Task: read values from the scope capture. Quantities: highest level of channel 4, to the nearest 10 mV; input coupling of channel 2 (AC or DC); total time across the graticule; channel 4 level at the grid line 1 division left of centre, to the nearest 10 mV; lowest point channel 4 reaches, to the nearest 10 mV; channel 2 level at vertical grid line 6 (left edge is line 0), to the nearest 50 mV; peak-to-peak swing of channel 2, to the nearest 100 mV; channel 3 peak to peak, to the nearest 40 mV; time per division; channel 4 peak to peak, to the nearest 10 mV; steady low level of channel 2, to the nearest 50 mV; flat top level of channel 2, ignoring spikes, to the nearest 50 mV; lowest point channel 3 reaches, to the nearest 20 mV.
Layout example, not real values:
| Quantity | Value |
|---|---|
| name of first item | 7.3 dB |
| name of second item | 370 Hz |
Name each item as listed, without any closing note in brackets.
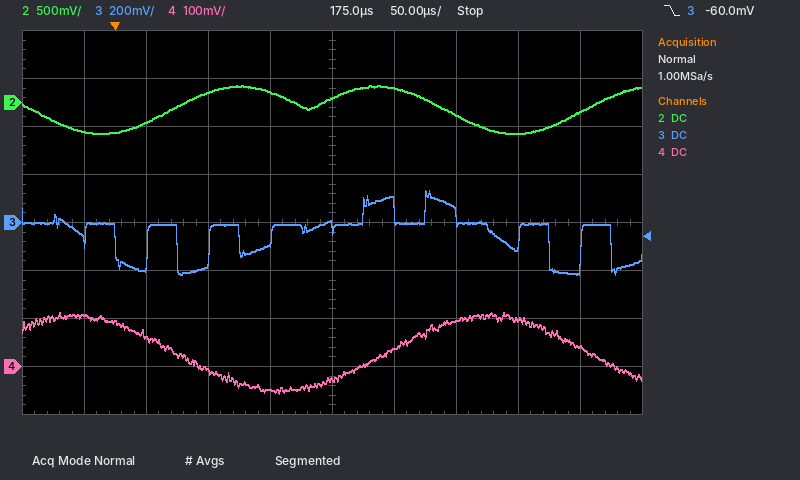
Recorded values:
| Quantity | Value |
|---|---|
| highest level of channel 4, to the nearest 10 mV | 110 mV |
| input coupling of channel 2 | DC |
| total time across the graticule | 500 µs |
| channel 4 level at the grid line 1 division left of centre, to the nearest 10 mV | -50 mV |
| lowest point channel 4 reaches, to the nearest 10 mV | -60 mV |
| channel 2 level at vertical grid line 6 (left edge is line 0), to the nearest 50 mV | 150 mV |
| peak-to-peak swing of channel 2, to the nearest 100 mV | 500 mV |
| channel 3 peak to peak, to the nearest 40 mV | 360 mV |
| time per division | 50 µs |
| channel 4 peak to peak, to the nearest 10 mV | 170 mV |
| steady low level of channel 2, to the nearest 50 mV | -300 mV |
| flat top level of channel 2, ignoring spikes, to the nearest 50 mV | 150 mV |
| lowest point channel 3 reaches, to the nearest 20 mV | -220 mV |
